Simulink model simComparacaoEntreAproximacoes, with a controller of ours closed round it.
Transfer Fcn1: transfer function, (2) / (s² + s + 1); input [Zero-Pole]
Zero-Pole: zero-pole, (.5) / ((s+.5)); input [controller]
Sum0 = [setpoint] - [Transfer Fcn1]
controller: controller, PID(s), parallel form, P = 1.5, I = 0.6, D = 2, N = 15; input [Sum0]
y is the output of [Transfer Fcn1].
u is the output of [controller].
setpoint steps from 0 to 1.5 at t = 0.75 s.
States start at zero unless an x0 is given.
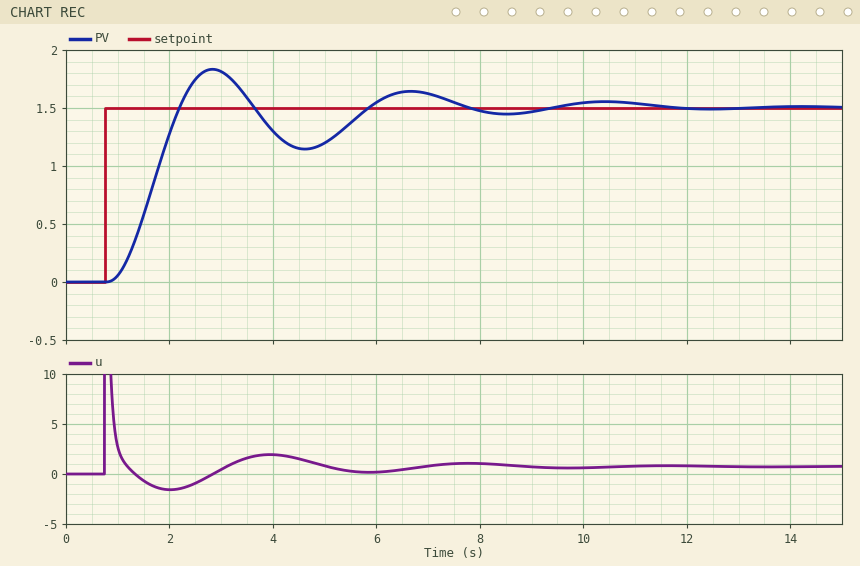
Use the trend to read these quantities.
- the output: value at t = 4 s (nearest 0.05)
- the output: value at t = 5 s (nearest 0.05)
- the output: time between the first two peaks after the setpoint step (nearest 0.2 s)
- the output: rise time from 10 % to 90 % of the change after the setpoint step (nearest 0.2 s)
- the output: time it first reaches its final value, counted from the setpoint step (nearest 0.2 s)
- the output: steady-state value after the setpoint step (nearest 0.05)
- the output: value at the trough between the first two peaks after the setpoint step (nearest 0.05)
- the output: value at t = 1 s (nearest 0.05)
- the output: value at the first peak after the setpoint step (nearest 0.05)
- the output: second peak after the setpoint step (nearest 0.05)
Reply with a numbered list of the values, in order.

1. 1.30
2. 1.20
3. 3.8 s
4. 1.0 s
5. 1.4 s
6. 1.50
7. 1.15
8. 0.05
9. 1.85
10. 1.65
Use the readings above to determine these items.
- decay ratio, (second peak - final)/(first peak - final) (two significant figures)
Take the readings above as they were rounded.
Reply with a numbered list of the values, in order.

1. 0.43
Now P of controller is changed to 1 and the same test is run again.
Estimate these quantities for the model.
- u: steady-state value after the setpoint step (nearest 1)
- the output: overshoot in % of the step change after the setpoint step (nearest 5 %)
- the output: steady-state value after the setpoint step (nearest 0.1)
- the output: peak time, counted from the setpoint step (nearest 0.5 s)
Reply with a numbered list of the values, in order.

1. 1
2. 10 %
3. 1.5
4. 2.0 s
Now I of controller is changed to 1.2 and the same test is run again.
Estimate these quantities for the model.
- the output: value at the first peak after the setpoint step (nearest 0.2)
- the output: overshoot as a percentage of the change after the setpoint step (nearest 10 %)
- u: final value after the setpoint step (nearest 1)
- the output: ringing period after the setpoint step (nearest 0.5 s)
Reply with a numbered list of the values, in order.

1. 2.0
2. 40 %
3. 1
4. 4.0 s
